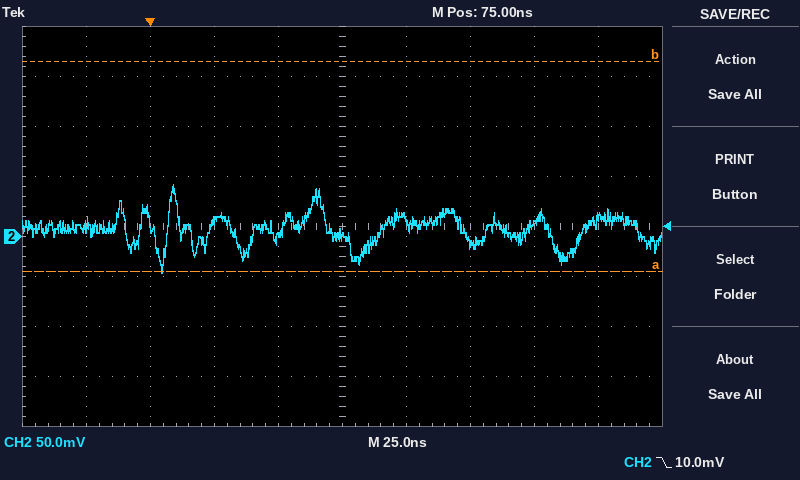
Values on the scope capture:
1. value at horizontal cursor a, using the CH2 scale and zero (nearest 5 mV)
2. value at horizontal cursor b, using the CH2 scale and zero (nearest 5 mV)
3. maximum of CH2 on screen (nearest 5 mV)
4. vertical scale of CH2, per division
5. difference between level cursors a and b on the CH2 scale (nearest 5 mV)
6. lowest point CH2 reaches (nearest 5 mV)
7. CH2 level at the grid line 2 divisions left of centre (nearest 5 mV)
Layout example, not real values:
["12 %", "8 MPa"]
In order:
["-35 mV", "175 mV", "50 mV", "50 mV", "210 mV", "-35 mV", "15 mV"]
